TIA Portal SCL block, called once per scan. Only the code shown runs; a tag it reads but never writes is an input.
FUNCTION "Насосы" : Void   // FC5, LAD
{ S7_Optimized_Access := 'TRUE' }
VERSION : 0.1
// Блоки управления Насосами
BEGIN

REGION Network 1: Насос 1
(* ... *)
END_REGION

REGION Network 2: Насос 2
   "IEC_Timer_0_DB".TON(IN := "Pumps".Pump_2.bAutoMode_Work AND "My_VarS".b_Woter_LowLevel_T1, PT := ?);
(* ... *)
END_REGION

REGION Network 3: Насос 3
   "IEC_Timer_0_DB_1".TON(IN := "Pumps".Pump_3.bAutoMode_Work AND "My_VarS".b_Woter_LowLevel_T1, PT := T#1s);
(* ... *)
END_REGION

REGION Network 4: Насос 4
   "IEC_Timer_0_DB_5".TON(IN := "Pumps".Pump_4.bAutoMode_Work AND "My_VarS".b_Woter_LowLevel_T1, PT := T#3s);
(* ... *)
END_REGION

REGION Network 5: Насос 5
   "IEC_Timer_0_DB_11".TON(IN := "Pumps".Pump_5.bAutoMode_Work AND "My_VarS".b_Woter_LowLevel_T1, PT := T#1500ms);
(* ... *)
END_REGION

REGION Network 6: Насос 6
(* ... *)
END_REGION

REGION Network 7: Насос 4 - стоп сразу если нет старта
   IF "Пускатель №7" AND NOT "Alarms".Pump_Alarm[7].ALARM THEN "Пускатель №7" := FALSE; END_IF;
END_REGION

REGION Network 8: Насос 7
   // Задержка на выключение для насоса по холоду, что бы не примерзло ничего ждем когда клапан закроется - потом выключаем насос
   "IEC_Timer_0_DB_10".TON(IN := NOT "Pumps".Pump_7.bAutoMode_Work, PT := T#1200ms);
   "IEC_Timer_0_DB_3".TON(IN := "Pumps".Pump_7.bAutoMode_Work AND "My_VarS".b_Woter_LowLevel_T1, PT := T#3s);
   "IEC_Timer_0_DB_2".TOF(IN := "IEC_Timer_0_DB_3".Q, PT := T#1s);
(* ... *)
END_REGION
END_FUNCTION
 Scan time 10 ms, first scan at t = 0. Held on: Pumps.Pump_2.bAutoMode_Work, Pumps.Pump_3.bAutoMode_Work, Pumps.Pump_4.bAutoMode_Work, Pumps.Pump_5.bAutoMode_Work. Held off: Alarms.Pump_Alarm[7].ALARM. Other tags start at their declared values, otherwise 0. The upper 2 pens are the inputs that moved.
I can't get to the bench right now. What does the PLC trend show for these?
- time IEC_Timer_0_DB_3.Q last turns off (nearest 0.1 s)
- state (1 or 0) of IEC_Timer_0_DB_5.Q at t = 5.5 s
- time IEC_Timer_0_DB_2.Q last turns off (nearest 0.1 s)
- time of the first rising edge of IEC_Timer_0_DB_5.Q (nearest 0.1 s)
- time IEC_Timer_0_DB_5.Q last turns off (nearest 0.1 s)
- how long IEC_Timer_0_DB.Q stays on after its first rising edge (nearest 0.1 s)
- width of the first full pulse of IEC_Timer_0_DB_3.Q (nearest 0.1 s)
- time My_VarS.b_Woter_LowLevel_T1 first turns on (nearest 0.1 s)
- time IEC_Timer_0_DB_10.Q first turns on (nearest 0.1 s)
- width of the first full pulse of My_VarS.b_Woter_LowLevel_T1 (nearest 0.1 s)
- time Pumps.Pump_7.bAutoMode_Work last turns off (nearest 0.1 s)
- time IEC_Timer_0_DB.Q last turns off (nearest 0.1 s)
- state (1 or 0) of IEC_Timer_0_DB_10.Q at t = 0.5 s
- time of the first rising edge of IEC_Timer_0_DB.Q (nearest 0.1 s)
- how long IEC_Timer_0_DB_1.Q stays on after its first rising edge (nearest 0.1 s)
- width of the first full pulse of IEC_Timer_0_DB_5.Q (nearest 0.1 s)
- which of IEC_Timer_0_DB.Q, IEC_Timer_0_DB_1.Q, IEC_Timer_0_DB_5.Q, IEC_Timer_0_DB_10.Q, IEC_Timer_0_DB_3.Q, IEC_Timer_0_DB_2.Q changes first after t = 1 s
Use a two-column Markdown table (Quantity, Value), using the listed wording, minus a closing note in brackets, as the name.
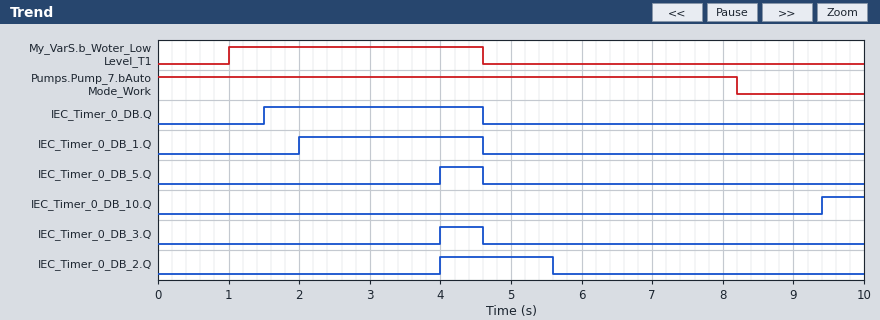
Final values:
| Quantity | Value |
|---|---|
| time IEC_Timer_0_DB_3.Q last turns off | 4.6 s |
| state (1 or 0) of IEC_Timer_0_DB_5.Q at t = 5.5 s | 0 |
| time IEC_Timer_0_DB_2.Q last turns off | 5.6 s |
| time of the first rising edge of IEC_Timer_0_DB_5.Q | 4.0 s |
| time IEC_Timer_0_DB_5.Q last turns off | 4.6 s |
| how long IEC_Timer_0_DB.Q stays on after its first rising edge | 3.1 s |
| width of the first full pulse of IEC_Timer_0_DB_3.Q | 0.6 s |
| time My_VarS.b_Woter_LowLevel_T1 first turns on | 1.0 s |
| time IEC_Timer_0_DB_10.Q first turns on | 9.4 s |
| width of the first full pulse of My_VarS.b_Woter_LowLevel_T1 | 3.6 s |
| time Pumps.Pump_7.bAutoMode_Work last turns off | 8.2 s |
| time IEC_Timer_0_DB.Q last turns off | 4.6 s |
| state (1 or 0) of IEC_Timer_0_DB_10.Q at t = 0.5 s | 0 |
| time of the first rising edge of IEC_Timer_0_DB.Q | 1.5 s |
| how long IEC_Timer_0_DB_1.Q stays on after its first rising edge | 2.6 s |
| width of the first full pulse of IEC_Timer_0_DB_5.Q | 0.6 s |
| which of IEC_Timer_0_DB.Q, IEC_Timer_0_DB_1.Q, IEC_Timer_0_DB_5.Q, IEC_Timer_0_DB_10.Q, IEC_Timer_0_DB_3.Q, IEC_Timer_0_DB_2.Q changes first after t = 1 s | IEC_Timer_0_DB.Q |
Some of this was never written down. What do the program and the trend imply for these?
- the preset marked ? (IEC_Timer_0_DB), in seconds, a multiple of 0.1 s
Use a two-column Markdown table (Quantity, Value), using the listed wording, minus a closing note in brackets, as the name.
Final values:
| Quantity | Value |
|---|---|
| the preset marked ? (IEC_Timer_0_DB), in seconds, a multiple of 0.1 s | 0.5 s |
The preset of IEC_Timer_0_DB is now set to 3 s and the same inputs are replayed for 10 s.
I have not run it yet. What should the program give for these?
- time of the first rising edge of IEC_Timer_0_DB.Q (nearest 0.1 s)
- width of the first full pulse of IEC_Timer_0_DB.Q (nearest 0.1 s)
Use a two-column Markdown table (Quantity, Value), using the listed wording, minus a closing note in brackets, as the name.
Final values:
| Quantity | Value |
|---|---|
| time of the first rising edge of IEC_Timer_0_DB.Q | 4.0 s |
| width of the first full pulse of IEC_Timer_0_DB.Q | 0.6 s |
